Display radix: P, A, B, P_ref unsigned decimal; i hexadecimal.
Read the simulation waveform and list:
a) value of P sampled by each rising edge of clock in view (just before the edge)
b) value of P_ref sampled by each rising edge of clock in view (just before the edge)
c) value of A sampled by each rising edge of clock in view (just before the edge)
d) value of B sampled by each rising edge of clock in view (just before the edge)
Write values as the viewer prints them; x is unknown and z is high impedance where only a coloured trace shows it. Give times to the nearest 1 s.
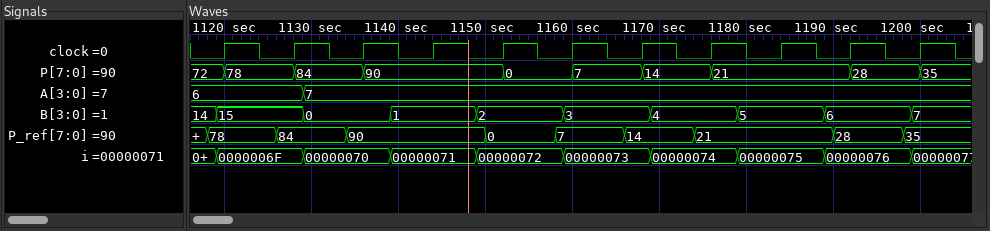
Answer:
72, 78, 84, 90, 90, 0, 7, 14, 21, 21, 28
78, 84, 90, 90, 0, 7, 14, 21, 21, 28, 35
6, 6, 7, 7, 7, 7, 7, 7, 7, 7, 7
15, 15, 0, 1, 2, 3, 3, 4, 5, 6, 7
